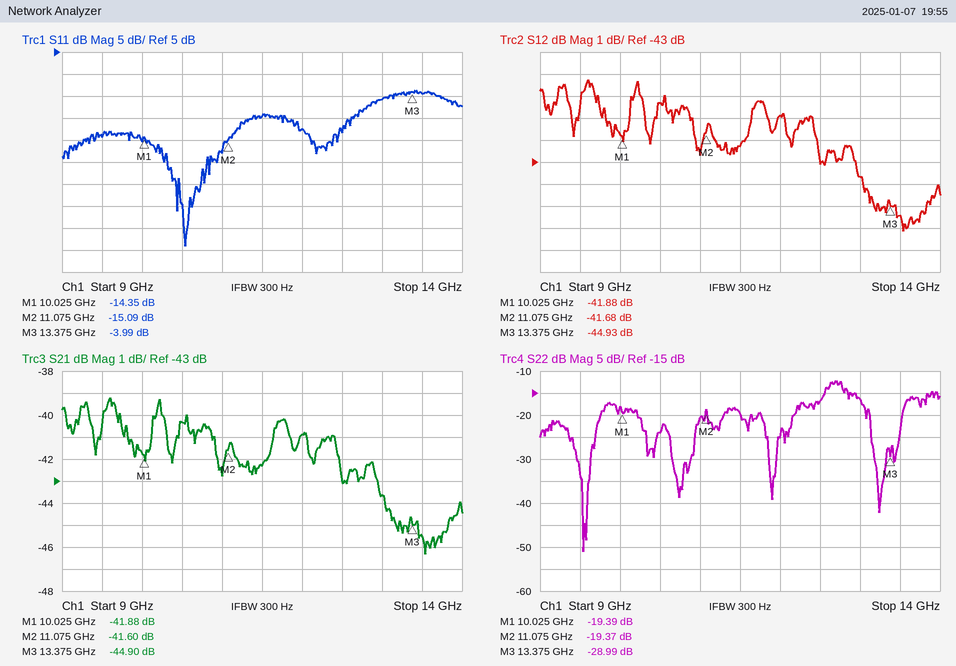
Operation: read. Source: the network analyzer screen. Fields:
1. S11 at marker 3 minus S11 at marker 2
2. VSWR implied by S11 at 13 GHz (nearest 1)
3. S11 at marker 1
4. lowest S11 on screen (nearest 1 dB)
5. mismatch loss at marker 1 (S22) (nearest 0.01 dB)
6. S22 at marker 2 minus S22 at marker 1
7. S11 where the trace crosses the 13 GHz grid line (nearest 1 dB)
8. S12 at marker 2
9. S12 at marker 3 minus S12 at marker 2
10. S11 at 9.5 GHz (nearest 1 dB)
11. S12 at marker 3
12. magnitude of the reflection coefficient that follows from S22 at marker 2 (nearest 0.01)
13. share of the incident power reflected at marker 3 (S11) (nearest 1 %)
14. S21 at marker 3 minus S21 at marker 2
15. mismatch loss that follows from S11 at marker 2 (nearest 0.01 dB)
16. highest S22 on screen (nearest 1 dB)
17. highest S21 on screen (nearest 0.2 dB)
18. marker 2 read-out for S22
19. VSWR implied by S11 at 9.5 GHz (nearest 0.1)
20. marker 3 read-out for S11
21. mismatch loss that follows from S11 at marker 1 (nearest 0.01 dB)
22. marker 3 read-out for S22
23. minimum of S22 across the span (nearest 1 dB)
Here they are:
11.10 dB
3
-14.35 dB
-39 dB
0.05 dB
0.02 dB
-6 dB
-41.68 dB
-3.25 dB
-14 dB
-44.93 dB
0.11
40 %
-3.30 dB
0.14 dB
-12 dB
-39.2 dB
-19.37 dB
1.5
-3.99 dB
0.16 dB
-28.99 dB
-51 dB
